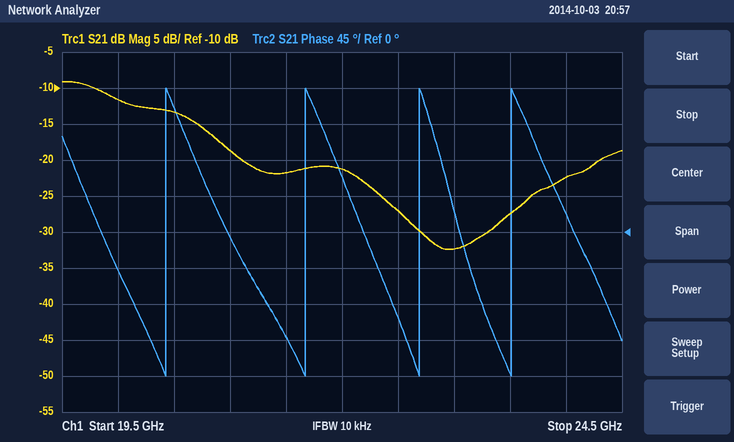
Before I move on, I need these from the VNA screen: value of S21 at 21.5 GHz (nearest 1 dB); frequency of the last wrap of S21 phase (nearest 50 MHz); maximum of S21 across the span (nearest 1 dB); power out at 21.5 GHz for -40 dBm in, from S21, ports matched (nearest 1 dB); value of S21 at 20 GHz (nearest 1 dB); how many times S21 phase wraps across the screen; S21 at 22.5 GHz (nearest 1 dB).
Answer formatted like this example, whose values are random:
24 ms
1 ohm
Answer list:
-22 dB
23.50 GHz
-9 dB
-62 dBm
-12 dB
4
-27 dB
